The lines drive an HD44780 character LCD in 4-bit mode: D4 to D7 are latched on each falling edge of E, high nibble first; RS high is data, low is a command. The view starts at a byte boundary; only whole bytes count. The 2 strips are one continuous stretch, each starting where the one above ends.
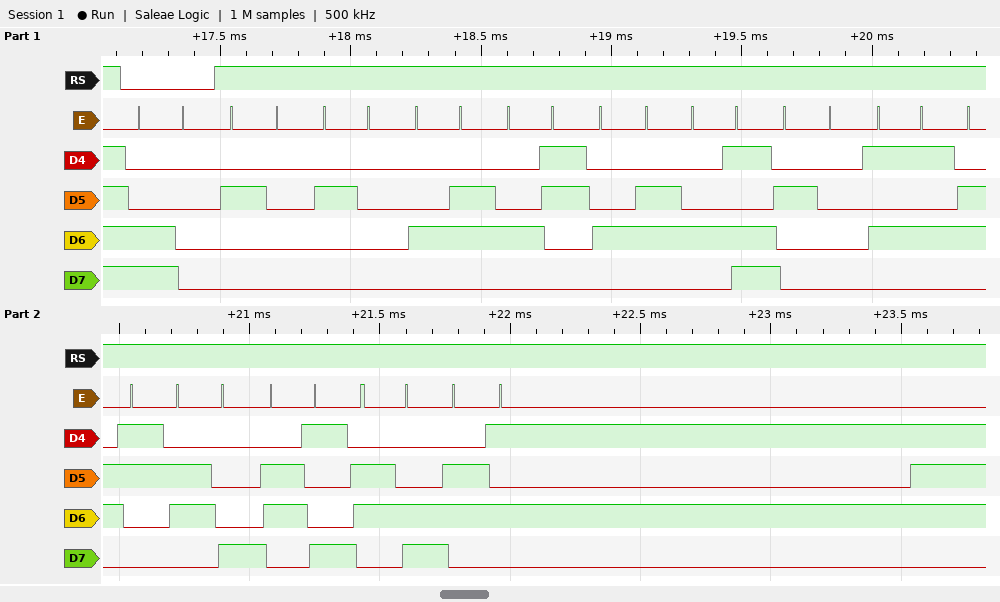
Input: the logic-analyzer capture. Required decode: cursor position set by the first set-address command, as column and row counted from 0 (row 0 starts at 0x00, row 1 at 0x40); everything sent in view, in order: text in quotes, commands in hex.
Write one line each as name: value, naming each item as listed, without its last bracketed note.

cursor position set by the first set-address command, as column and row counted from 0: column 0, row 1
everything sent in view, in order: text in quotes, commands in hex: 0xC0 "  FCFM Uchile"
